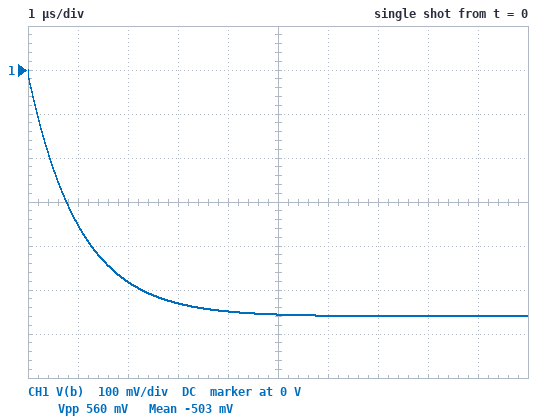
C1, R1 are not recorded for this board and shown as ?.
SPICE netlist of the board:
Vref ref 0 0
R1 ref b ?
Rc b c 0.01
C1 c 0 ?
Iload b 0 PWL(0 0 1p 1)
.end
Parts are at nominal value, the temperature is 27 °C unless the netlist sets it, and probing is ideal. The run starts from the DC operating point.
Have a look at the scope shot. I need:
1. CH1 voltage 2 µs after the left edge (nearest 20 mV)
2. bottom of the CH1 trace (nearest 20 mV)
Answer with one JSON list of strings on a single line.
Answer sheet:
["-480 mV", "-560 mV"]
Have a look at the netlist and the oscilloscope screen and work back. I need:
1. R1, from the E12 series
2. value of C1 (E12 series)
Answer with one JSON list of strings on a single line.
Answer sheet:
["0.56 Ω", "1.8 µF"]
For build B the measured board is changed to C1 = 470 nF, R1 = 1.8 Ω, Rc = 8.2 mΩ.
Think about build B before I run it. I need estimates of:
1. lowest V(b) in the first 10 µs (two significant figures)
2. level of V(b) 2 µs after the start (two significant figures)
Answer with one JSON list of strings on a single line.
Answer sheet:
["-1.8 V", "-1.6 V"]
